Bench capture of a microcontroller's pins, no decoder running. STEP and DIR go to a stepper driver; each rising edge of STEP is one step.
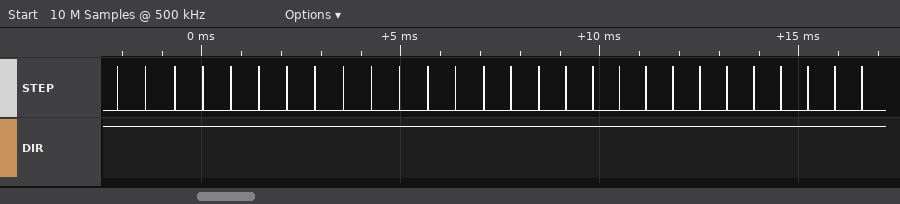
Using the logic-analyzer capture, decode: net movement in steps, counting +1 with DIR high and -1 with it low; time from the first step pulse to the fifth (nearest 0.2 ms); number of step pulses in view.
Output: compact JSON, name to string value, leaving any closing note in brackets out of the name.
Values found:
{"net movement in steps, counting +1 with DIR high and -1 with it low": "+28", "time from the first step pulse to the fifth": "2.8 ms", "number of step pulses in view": "28"}
